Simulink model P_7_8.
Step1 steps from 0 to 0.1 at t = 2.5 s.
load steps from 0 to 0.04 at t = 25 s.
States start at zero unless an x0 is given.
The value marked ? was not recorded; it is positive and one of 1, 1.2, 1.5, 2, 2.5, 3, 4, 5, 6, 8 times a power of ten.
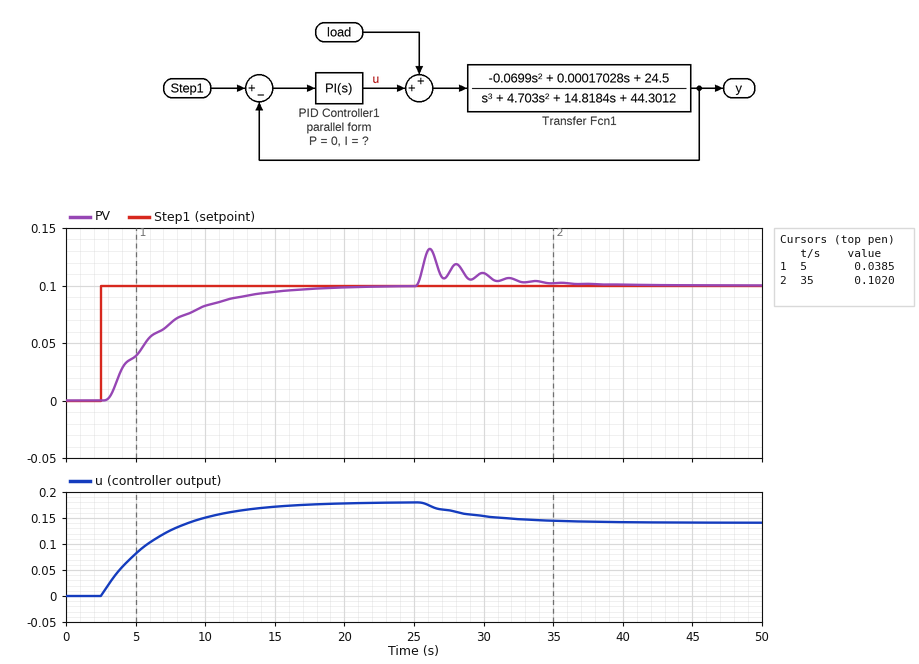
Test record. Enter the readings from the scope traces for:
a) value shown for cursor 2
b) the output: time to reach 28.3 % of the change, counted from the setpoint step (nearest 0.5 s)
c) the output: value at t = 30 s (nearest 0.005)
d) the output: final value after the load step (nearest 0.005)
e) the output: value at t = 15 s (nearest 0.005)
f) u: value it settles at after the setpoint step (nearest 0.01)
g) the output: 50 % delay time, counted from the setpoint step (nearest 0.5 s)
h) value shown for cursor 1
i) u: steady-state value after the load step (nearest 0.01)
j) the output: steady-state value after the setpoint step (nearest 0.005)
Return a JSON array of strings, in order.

["0.1020", "1.5 s", "0.110", "0.100", "0.095", "0.18", "3.0 s", "0.0385", "0.14", "0.100"]
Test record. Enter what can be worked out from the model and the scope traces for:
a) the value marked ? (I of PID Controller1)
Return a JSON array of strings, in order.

["0.4"]
